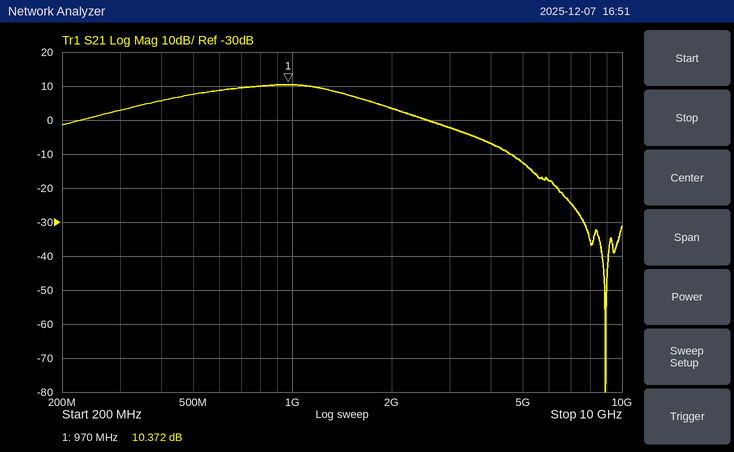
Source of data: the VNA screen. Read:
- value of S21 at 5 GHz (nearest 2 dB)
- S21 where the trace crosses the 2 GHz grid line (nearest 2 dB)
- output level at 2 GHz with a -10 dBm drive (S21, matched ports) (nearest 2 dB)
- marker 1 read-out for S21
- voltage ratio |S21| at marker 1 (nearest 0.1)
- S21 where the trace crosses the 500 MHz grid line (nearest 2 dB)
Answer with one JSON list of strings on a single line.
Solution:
["-12 dB", "4 dB", "-6 dBm", "10.372 dB", "3.3", "8 dB"]
